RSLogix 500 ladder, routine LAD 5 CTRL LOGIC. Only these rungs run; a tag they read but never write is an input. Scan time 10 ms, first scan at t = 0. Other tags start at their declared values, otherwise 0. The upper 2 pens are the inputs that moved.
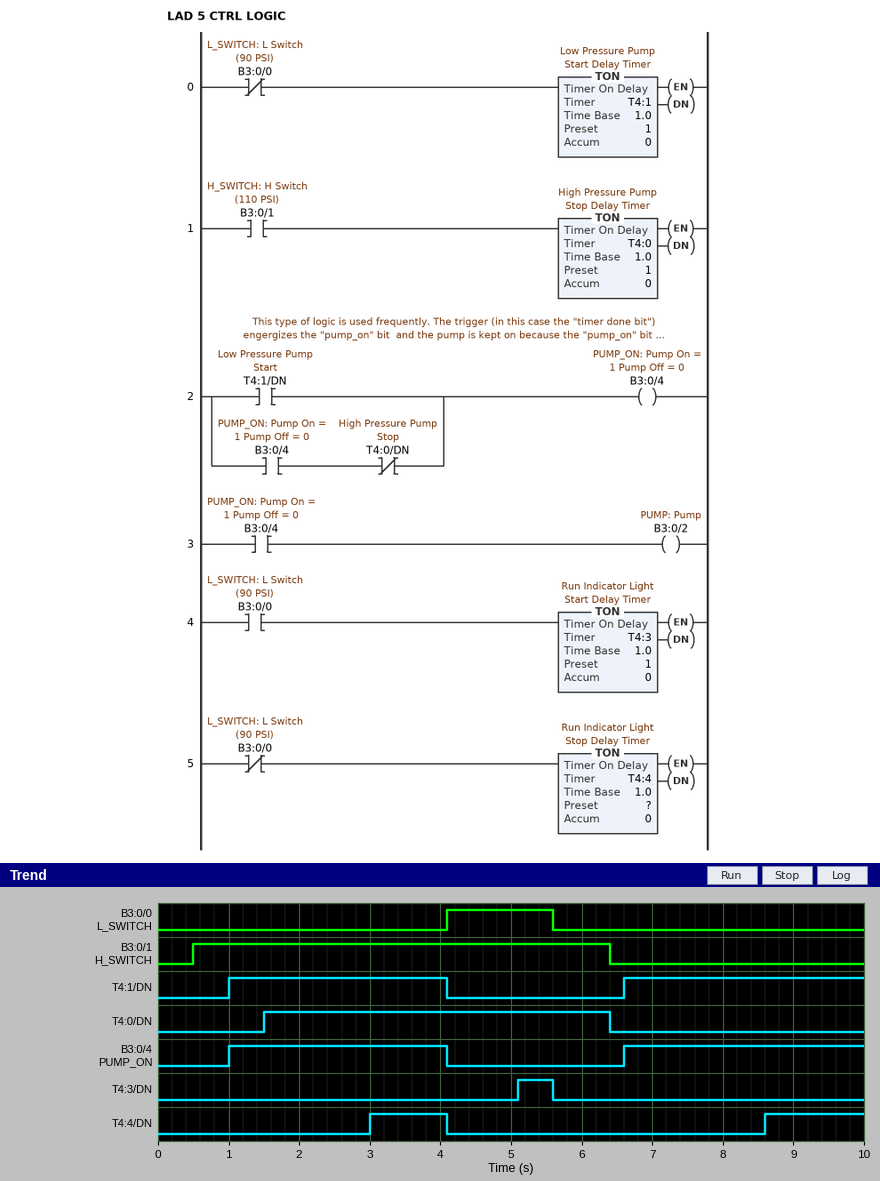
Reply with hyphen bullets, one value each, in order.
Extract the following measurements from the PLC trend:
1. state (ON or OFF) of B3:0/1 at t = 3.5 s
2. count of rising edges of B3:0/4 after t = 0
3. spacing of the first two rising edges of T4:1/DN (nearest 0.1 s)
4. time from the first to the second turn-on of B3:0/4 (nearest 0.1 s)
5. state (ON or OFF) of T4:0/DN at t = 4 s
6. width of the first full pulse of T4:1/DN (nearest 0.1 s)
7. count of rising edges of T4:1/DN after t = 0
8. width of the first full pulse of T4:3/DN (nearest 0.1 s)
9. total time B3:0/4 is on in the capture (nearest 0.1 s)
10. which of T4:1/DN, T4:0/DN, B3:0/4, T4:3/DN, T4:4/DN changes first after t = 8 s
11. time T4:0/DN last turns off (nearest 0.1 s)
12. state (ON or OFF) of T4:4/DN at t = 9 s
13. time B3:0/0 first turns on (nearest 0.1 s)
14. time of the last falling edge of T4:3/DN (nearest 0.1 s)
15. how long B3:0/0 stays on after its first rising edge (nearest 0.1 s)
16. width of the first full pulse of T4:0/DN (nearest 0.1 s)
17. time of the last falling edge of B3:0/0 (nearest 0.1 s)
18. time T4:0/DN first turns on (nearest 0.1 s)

- ON
- 2
- 5.6 s
- 5.6 s
- ON
- 3.1 s
- 2
- 0.5 s
- 6.5 s
- T4:4/DN
- 6.4 s
- ON
- 4.1 s
- 5.6 s
- 1.5 s
- 4.9 s
- 5.6 s
- 1.5 s
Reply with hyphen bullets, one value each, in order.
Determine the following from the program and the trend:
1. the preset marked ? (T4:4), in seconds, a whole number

- 3 s
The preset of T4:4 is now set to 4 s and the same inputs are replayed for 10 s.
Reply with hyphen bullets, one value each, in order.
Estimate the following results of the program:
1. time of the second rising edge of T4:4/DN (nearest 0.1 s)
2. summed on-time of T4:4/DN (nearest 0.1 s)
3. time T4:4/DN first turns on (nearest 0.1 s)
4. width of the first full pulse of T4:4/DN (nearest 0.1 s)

- 9.6 s
- 0.5 s
- 4.0 s
- 0.1 s
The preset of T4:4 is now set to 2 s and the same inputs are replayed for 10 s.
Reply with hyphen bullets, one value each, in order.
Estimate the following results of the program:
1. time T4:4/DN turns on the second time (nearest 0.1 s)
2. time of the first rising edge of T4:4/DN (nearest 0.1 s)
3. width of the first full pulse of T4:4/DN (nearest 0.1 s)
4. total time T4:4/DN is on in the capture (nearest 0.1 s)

- 7.6 s
- 2.0 s
- 2.1 s
- 4.5 s
